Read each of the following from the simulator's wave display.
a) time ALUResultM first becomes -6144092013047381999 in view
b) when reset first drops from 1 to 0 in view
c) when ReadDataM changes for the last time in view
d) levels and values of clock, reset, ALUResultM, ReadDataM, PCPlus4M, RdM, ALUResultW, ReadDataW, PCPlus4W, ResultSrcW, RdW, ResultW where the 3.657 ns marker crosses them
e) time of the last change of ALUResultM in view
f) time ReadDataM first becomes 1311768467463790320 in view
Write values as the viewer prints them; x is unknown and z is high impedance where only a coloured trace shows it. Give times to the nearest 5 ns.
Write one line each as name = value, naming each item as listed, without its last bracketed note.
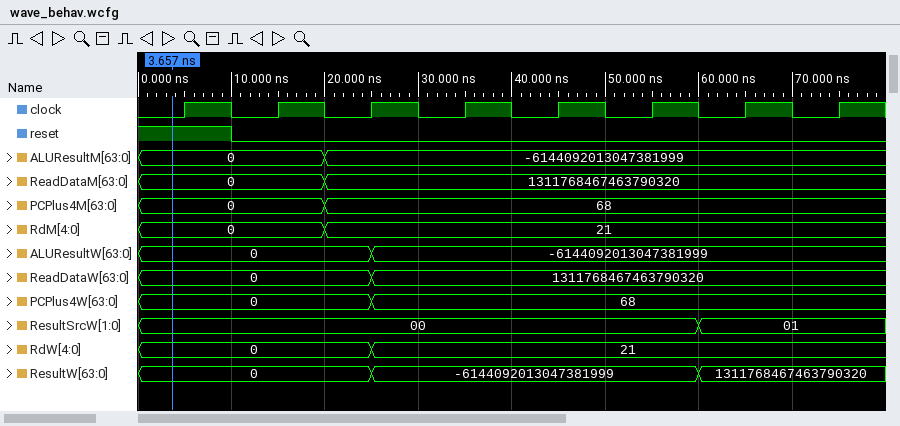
time ALUResultM first becomes -6144092013047381999 in view = 20 ns
when reset first drops from 1 to 0 in view = 10 ns
when ReadDataM changes for the last time in view = 20 ns
levels and values of clock, reset, ALUResultM, ReadDataM, PCPlus4M, RdM, ALUResultW, ReadDataW, PCPlus4W, ResultSrcW, RdW, ResultW where the 3.657 ns marker crosses them = clock=0, reset=1, ALUResultM=0, ReadDataM=0, PCPlus4M=0, RdM=0, ALUResultW=0, ReadDataW=0, PCPlus4W=0, ResultSrcW=00, RdW=0, ResultW=0
time of the last change of ALUResultM in view = 20 ns
time ReadDataM first becomes 1311768467463790320 in view = 20 ns
